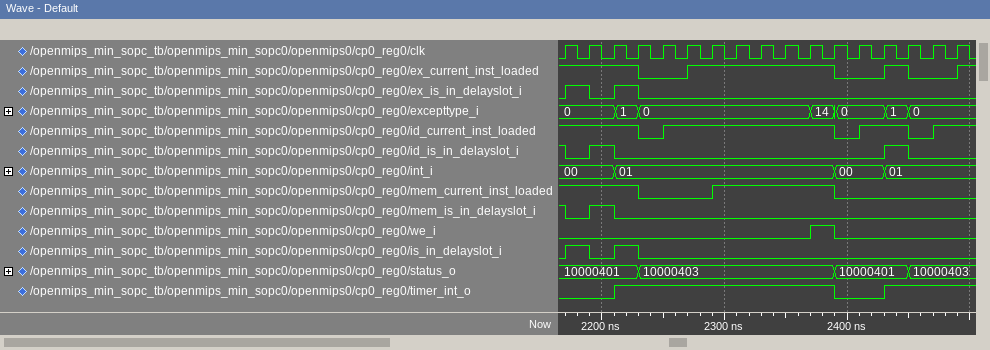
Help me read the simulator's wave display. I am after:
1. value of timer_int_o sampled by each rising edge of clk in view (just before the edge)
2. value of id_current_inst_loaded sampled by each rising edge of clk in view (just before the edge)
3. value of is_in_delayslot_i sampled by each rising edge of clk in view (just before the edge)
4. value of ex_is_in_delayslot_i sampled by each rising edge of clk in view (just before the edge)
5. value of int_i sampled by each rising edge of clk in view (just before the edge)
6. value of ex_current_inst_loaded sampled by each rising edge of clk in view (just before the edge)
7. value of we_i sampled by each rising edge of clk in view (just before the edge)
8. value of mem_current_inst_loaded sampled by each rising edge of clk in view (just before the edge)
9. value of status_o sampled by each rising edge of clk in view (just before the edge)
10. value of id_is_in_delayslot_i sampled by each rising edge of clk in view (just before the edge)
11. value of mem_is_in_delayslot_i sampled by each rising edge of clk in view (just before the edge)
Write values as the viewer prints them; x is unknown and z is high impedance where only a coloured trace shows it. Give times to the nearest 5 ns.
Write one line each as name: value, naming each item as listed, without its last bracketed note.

value of timer_int_o sampled by each rising edge of clk in view: 0 0 0 1 1 1 1 1 1 1 1 1 0 0 1 1 1
value of id_current_inst_loaded sampled by each rising edge of clk in view: 1 1 1 1 0 1 1 1 1 1 1 1 0 1 1 0 1
value of is_in_delayslot_i sampled by each rising edge of clk in view: 0 1 0 1 0 0 0 0 0 0 0 0 0 0 0 0 0
value of ex_is_in_delayslot_i sampled by each rising edge of clk in view: 0 1 0 1 0 0 0 0 0 0 0 0 0 0 0 0 0
value of int_i sampled by each rising edge of clk in view: 00, 00, 00, 01, 01, 01, 01, 01, 01, 01, 01, 01, 00, 00, 01, 01, 01
value of ex_current_inst_loaded sampled by each rising edge of clk in view: 1 1 1 1 0 0 1 1 1 1 1 1 0 0 1 0 0
value of we_i sampled by each rising edge of clk in view: 0 0 0 0 0 0 0 0 0 0 0 1 0 0 0 0 0
value of mem_current_inst_loaded sampled by each rising edge of clk in view: 1 1 1 1 0 0 0 1 1 1 1 1 0 0 0 0 0
value of status_o sampled by each rising edge of clk in view: 10000401, 10000401, 10000401, 10000401, 10000403, 10000403, 10000403, 10000403, 10000403, 10000403, 10000403, 10000403, 10000401, 10000401, 10000401, 10000403, 10000403
value of id_is_in_delayslot_i sampled by each rising edge of clk in view: 1 0 1 0 0 0 0 0 0 0 0 0 0 0 1 0 0
value of mem_is_in_delayslot_i sampled by each rising edge of clk in view: 1 0 1 0 0 0 0 0 0 0 0 0 0 0 0 0 0
